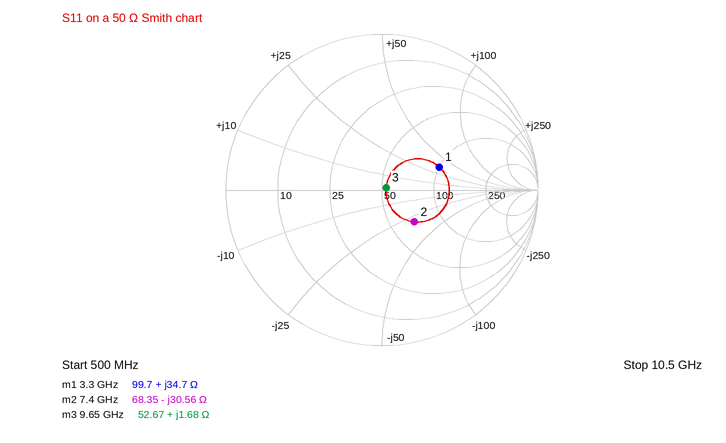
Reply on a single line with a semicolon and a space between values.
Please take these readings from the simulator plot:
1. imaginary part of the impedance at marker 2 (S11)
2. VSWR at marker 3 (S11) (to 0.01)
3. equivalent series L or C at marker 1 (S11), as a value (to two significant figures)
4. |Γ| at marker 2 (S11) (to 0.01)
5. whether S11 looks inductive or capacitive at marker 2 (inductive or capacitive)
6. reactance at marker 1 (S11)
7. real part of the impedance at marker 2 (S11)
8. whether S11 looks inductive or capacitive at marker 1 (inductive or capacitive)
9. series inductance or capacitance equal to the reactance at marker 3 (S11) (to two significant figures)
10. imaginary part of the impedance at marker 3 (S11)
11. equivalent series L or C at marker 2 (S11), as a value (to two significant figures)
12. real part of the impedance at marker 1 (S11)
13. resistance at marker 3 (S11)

-30.56 Ω; 1.06; 1.7 nH; 0.29; capacitive; +34.7 Ω; 68.35 Ω; inductive; 28 pH; +1.68 Ω; 700 fF; 99.7 Ω; 52.67 Ω
